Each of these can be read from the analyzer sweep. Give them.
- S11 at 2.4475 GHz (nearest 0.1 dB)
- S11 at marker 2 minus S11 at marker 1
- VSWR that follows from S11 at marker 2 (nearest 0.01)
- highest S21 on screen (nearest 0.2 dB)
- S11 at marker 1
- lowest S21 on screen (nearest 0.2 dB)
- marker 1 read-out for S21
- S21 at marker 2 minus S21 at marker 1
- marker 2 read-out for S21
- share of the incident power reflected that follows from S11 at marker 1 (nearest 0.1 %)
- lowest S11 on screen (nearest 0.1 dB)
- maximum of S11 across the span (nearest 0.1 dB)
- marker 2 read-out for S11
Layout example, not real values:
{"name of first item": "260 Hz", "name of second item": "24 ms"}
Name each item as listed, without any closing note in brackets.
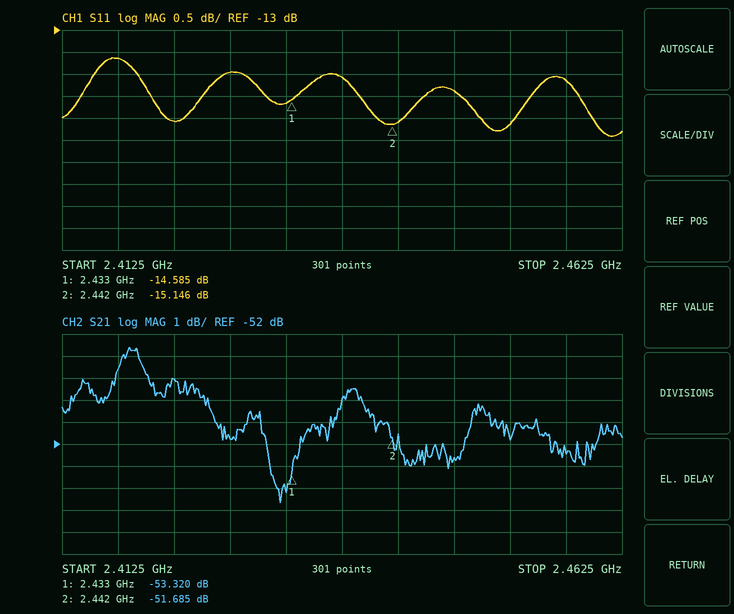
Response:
{"S11 at 2.4475 GHz": "-14.4 dB", "S11 at marker 2 minus S11 at marker 1": "-0.561 dB", "VSWR that follows from S11 at marker 2": "1.42", "highest S21 on screen": "-47.6 dB", "S11 at marker 1": "-14.585 dB", "lowest S21 on screen": "-54.6 dB", "marker 1 read-out for S21": "-53.320 dB", "S21 at marker 2 minus S21 at marker 1": "1.635 dB", "marker 2 read-out for S21": "-51.685 dB", "share of the incident power reflected that follows from S11 at marker 1": "3.5 %", "lowest S11 on screen": "-15.4 dB", "maximum of S11 across the span": "-13.6 dB", "marker 2 read-out for S11": "-15.146 dB"}
